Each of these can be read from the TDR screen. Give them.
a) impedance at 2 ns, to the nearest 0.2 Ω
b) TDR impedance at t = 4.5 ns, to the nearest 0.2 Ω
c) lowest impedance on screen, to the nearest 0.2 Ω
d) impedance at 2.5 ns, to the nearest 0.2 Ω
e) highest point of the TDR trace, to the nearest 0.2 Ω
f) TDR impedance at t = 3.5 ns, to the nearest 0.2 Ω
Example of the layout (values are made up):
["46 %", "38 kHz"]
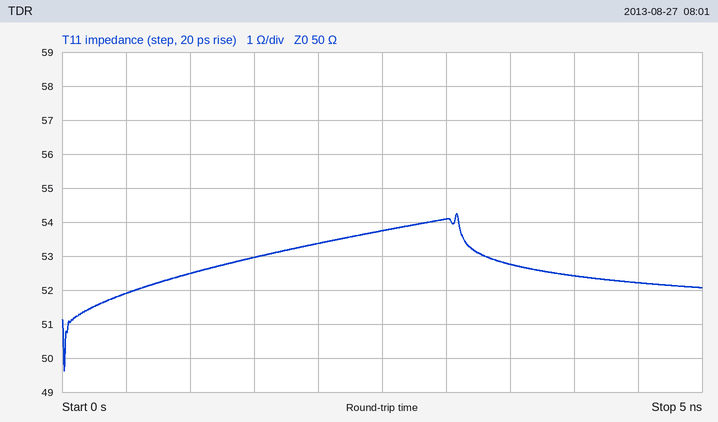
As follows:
["53.4 Ω", "52.2 Ω", "49.6 Ω", "53.8 Ω", "54.2 Ω", "52.8 Ω"]
